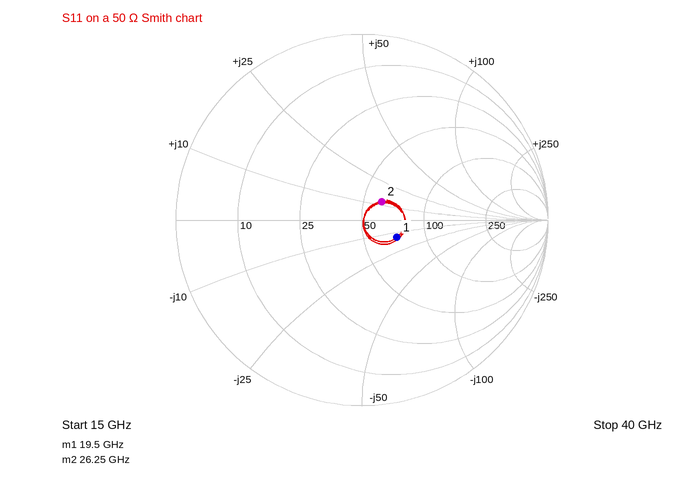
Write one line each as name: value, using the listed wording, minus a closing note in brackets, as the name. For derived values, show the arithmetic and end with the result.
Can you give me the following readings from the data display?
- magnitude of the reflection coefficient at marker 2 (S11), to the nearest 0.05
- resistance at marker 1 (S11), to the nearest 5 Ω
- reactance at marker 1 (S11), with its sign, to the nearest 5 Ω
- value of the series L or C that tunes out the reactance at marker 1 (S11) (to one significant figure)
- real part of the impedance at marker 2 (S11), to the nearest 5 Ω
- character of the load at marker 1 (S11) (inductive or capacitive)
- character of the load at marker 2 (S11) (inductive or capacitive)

magnitude of the reflection coefficient at marker 2 (S11), to the nearest 0.05: 0.15
resistance at marker 1 (S11), to the nearest 5 Ω: 70 Ω
reactance at marker 1 (S11), with its sign, to the nearest 5 Ω: -15 Ω
value of the series L or C that tunes out the reactance at marker 1 (S11): L = 15 Ω/(2π × 19.5 GHz) ≈ 122 pH, so 100 pH to one significant figure
real part of the impedance at marker 2 (S11), to the nearest 5 Ω: 60 Ω
character of the load at marker 1 (S11): capacitive
character of the load at marker 2 (S11): inductive
